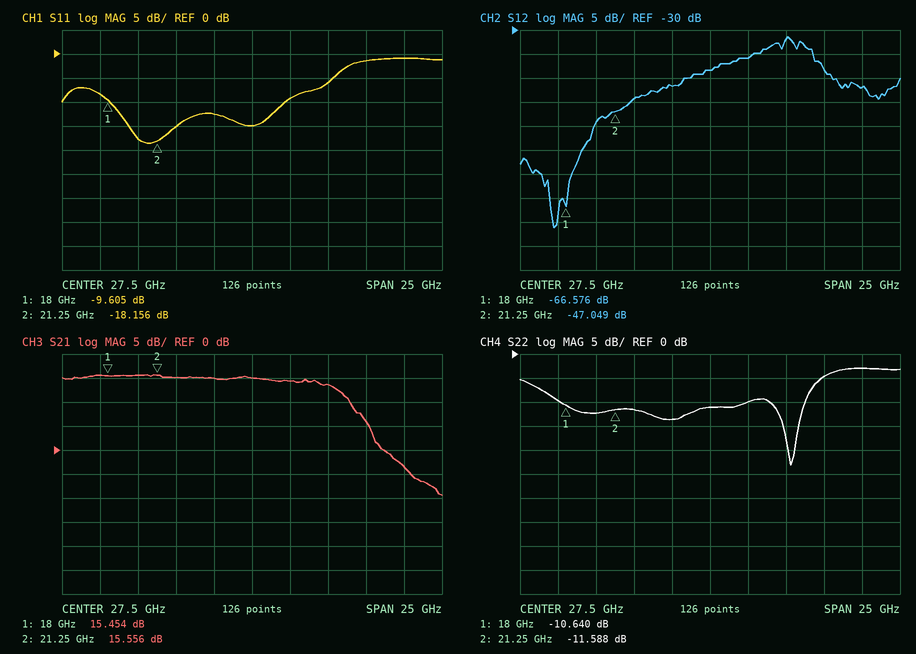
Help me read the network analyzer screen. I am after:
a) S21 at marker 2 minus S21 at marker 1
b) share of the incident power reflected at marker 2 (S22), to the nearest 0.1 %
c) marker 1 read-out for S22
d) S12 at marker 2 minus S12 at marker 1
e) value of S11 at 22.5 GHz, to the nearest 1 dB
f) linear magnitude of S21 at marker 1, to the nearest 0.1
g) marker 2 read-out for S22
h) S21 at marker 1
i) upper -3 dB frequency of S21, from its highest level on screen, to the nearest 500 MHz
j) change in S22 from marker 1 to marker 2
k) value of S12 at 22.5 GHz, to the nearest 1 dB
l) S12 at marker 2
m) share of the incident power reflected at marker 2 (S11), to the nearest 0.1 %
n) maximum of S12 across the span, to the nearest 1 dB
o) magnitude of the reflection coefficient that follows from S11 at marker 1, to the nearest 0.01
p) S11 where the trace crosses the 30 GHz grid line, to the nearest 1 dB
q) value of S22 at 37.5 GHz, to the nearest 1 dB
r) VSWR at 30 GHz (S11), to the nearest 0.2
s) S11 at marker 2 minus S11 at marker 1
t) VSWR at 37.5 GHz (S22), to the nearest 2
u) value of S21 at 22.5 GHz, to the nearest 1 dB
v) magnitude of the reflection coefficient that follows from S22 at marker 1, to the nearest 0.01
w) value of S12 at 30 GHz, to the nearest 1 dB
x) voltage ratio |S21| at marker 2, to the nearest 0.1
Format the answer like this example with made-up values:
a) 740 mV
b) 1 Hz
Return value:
a) 0.102 dB
b) 6.9 %
c) -10.640 dB
d) 19.527 dB
e) -15 dB
f) 5.9
g) -11.588 dB
h) 15.454 dB
i) 33.0 GHz
j) -0.948 dB
k) -44 dB
l) -47.049 dB
m) 1.5 %
n) -31 dB
o) 0.33
p) -9 dB
q) -3 dB
r) 2.0
s) -8.551 dB
t) 6
u) 15 dB
v) 0.29
w) -36 dB
x) 6.0
